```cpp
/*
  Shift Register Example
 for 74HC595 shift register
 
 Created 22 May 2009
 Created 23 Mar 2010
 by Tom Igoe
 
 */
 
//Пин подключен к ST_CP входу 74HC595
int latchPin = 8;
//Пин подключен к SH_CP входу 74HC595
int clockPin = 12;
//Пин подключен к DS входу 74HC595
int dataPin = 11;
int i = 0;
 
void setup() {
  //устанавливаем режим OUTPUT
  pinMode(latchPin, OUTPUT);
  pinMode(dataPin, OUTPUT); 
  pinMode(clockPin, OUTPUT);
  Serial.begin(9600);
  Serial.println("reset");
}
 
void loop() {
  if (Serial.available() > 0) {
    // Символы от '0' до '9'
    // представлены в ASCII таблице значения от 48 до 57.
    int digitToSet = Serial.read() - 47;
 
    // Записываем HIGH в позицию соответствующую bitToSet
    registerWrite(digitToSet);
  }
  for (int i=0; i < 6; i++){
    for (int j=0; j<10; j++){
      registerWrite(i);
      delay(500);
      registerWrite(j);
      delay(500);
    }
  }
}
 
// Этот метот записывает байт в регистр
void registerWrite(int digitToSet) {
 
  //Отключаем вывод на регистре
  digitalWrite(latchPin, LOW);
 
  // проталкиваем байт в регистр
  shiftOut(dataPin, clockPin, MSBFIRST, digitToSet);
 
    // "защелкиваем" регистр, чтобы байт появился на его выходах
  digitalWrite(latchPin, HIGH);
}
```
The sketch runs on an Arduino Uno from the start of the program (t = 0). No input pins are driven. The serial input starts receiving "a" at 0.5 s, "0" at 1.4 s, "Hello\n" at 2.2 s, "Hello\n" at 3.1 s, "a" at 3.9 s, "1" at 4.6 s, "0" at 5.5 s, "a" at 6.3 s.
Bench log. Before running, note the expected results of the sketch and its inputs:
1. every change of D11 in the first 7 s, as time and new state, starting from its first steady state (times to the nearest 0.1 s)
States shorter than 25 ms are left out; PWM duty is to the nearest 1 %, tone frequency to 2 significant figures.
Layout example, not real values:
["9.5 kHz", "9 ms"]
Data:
["0 s low; 1.5 s high; 2 s low; 3.5 s high; 4 s low; 5.5 s high; 6 s low"]
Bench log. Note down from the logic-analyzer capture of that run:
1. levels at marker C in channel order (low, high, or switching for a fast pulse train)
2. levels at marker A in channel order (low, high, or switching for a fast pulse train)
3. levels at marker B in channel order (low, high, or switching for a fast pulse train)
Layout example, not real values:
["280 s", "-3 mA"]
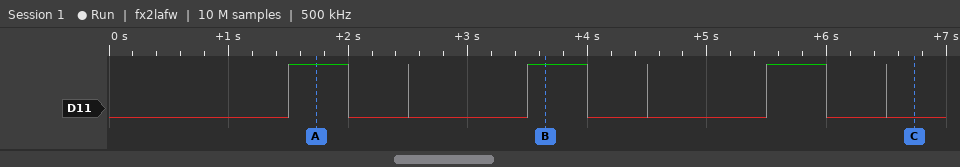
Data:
["D11 low", "D11 high", "D11 high"]
